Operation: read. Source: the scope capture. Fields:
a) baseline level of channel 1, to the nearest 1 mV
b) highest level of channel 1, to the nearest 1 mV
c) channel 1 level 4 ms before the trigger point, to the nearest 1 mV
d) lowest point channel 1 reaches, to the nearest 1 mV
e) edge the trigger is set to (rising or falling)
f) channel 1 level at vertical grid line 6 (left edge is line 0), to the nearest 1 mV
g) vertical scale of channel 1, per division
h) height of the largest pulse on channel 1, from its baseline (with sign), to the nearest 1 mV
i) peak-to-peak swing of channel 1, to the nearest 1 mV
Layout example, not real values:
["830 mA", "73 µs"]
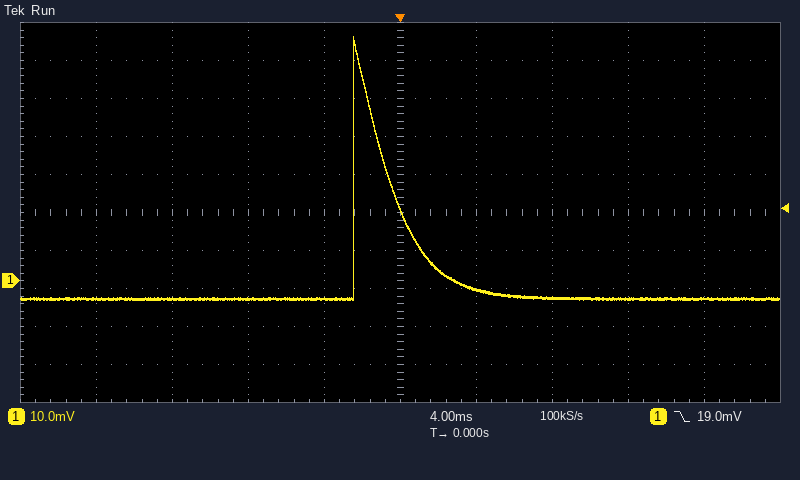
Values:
["-5 mV", "64 mV", "-5 mV", "-5 mV", "falling", "-2 mV", "10 mV", "+69 mV", "69 mV"]
